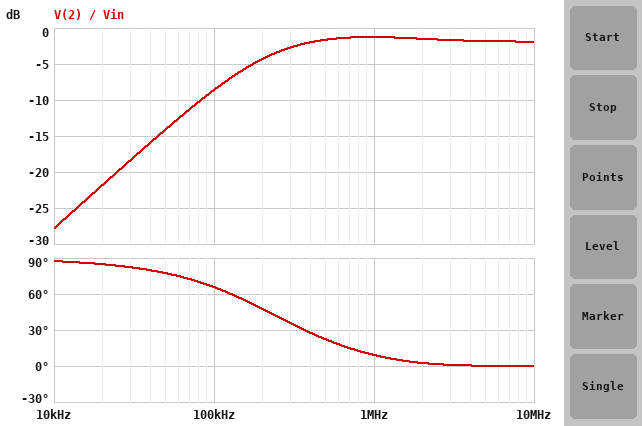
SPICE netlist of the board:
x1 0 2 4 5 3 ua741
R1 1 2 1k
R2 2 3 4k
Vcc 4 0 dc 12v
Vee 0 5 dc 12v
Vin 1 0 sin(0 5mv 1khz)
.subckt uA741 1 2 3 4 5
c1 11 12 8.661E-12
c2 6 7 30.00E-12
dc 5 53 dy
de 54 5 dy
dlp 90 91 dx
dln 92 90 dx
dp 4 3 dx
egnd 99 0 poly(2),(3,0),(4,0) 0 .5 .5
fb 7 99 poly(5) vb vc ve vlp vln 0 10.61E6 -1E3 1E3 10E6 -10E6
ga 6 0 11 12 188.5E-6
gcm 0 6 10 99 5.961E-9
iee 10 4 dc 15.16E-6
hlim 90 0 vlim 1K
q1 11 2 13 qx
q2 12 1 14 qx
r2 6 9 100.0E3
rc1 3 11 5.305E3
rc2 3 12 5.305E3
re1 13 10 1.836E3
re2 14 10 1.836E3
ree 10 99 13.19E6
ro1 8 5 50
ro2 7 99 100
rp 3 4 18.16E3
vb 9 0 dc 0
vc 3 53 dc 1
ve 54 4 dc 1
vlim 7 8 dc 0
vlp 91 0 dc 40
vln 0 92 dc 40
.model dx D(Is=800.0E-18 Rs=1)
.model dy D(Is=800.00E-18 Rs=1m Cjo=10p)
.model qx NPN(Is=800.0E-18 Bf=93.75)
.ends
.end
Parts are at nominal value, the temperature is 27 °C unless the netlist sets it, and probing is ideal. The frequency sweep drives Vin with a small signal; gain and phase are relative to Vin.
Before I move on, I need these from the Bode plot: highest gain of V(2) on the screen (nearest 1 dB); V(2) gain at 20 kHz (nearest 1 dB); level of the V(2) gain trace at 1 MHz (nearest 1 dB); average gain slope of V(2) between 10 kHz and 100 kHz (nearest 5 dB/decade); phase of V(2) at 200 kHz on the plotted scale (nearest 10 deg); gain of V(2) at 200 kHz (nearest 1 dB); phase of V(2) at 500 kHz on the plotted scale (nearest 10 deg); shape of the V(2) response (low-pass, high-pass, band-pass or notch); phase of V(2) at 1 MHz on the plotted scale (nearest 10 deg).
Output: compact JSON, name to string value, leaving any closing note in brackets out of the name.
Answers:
{"highest gain of V(2) on the screen": "-1 dB", "V(2) gain at 20 kHz": "-22 dB", "level of the V(2) gain trace at 1 MHz": "-1 dB", "average gain slope of V(2) between 10 kHz and 100 kHz": "20 dB/decade", "phase of V(2) at 200 kHz on the plotted scale": "50 deg", "gain of V(2) at 200 kHz": "-4 dB", "phase of V(2) at 500 kHz on the plotted scale": "20 deg", "shape of the V(2) response": "high-pass", "phase of V(2) at 1 MHz on the plotted scale": "10 deg"}
